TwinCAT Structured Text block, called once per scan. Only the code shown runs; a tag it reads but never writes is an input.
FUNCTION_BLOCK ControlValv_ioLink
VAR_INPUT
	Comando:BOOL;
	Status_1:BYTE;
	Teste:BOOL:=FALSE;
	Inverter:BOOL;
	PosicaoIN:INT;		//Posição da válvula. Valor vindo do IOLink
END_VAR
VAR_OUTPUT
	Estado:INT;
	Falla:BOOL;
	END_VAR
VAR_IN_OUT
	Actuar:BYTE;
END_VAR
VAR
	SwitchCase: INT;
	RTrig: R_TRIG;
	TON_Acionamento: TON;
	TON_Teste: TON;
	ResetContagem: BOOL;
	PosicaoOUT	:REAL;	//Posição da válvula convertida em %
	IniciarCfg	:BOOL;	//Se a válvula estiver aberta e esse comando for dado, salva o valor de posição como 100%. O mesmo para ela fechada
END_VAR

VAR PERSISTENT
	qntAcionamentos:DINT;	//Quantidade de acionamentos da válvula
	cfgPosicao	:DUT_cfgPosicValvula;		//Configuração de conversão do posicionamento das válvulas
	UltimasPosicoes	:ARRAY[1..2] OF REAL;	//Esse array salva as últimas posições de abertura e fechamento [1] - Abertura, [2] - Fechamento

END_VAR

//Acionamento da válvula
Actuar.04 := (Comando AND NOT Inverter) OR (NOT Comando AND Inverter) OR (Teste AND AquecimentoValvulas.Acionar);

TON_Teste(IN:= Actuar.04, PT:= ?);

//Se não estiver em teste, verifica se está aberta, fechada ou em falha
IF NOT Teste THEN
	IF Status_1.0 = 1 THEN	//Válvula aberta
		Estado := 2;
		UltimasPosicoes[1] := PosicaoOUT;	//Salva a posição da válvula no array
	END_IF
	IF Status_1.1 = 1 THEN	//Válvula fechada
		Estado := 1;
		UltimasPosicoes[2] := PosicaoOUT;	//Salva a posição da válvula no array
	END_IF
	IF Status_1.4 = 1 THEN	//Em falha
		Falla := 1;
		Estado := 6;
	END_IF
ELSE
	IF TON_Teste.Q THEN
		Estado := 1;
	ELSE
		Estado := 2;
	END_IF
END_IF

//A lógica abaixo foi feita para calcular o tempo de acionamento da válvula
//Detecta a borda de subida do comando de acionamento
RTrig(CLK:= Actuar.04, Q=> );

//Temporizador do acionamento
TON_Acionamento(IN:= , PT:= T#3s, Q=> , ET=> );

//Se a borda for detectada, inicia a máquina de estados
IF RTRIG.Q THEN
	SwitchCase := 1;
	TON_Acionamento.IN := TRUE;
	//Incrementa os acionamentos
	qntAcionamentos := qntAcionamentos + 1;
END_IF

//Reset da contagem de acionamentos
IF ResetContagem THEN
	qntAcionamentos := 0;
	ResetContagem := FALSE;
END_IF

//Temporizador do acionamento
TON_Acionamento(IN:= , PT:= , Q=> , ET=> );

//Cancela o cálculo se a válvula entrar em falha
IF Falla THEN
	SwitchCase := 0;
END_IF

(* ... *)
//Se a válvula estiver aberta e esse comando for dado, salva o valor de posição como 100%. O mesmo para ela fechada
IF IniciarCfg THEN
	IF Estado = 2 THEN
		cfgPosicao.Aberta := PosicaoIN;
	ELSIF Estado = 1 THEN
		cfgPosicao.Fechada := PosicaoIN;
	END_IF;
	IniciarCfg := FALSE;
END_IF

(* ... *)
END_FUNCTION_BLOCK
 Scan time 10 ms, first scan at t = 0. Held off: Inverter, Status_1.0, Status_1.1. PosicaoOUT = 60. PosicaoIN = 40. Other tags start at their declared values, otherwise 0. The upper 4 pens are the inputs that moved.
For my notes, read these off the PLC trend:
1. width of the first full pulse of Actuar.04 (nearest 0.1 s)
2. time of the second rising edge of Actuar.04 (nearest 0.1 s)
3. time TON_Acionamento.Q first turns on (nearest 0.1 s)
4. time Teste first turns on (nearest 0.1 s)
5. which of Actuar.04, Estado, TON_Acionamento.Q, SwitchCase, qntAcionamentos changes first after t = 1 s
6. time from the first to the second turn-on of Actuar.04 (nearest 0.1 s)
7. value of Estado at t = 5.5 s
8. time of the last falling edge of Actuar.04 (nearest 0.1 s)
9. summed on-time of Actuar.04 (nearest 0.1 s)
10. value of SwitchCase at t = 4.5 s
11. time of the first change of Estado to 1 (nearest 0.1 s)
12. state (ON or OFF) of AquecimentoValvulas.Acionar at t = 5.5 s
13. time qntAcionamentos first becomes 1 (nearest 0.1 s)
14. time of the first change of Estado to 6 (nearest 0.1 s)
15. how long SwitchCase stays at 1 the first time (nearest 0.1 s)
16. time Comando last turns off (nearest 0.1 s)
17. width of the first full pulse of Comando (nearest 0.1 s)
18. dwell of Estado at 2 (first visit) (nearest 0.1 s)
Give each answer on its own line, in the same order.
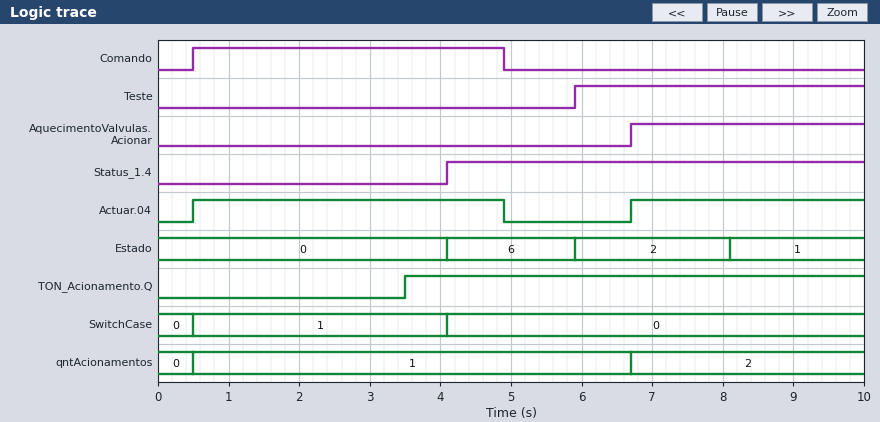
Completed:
4.4 s
6.7 s
3.5 s
5.9 s
TON_Acionamento.Q
6.2 s
6
4.9 s
7.7 s
0
8.1 s
OFF
0.5 s
4.1 s
3.6 s
4.9 s
4.4 s
2.2 s
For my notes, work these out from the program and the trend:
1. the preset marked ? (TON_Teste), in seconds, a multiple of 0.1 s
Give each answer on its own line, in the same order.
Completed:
1.4 s
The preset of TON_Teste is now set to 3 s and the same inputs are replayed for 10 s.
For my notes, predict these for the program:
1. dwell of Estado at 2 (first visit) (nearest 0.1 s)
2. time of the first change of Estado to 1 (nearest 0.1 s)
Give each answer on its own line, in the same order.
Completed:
3.8 s
9.7 s
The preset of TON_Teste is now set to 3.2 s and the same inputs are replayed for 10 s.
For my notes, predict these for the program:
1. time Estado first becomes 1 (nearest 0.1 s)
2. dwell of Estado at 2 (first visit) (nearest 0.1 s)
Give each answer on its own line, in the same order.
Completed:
9.9 s
4.0 s
